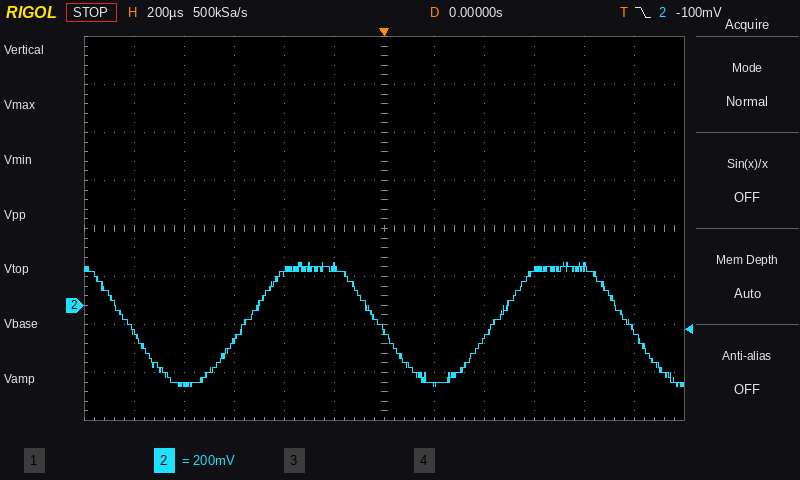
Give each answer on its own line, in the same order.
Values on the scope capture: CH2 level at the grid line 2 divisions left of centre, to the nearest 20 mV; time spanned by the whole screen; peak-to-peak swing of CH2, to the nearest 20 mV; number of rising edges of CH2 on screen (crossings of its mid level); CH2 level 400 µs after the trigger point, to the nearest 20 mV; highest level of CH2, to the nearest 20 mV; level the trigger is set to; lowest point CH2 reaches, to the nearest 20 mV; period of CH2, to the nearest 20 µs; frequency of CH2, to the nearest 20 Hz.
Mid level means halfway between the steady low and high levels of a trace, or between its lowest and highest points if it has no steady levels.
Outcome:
140 mV
2.4 ms
520 mV
2
-140 mV
180 mV
-100 mV
-340 mV
1.00 ms
1.00 kHz
